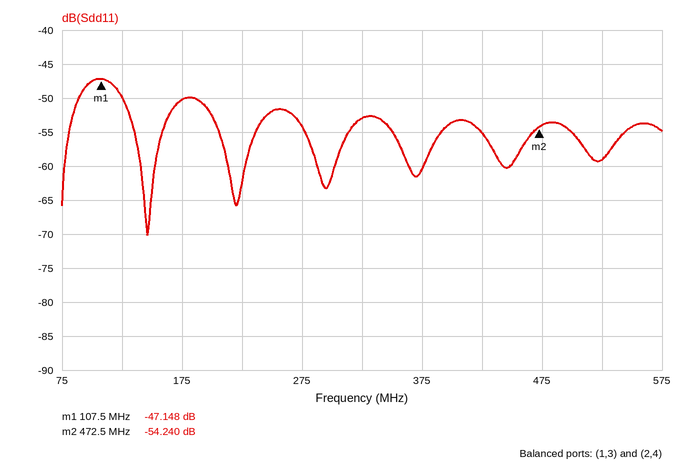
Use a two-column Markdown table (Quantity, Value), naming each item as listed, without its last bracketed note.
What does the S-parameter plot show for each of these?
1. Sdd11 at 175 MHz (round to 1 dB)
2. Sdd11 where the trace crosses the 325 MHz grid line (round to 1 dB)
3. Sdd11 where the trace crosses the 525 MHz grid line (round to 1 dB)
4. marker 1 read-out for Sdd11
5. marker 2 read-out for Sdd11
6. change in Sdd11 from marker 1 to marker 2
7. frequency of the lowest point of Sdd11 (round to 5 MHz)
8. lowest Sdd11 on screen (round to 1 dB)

| Quantity | Value |
|---|---|
| Sdd11 at 175 MHz | -50 dB |
| Sdd11 where the trace crosses the 325 MHz grid line | -53 dB |
| Sdd11 where the trace crosses the 525 MHz grid line | -59 dB |
| marker 1 read-out for Sdd11 | -47.148 dB |
| marker 2 read-out for Sdd11 | -54.240 dB |
| change in Sdd11 from marker 1 to marker 2 | -7.092 dB |
| frequency of the lowest point of Sdd11 | 145 MHz |
| lowest Sdd11 on screen | -70 dB |
